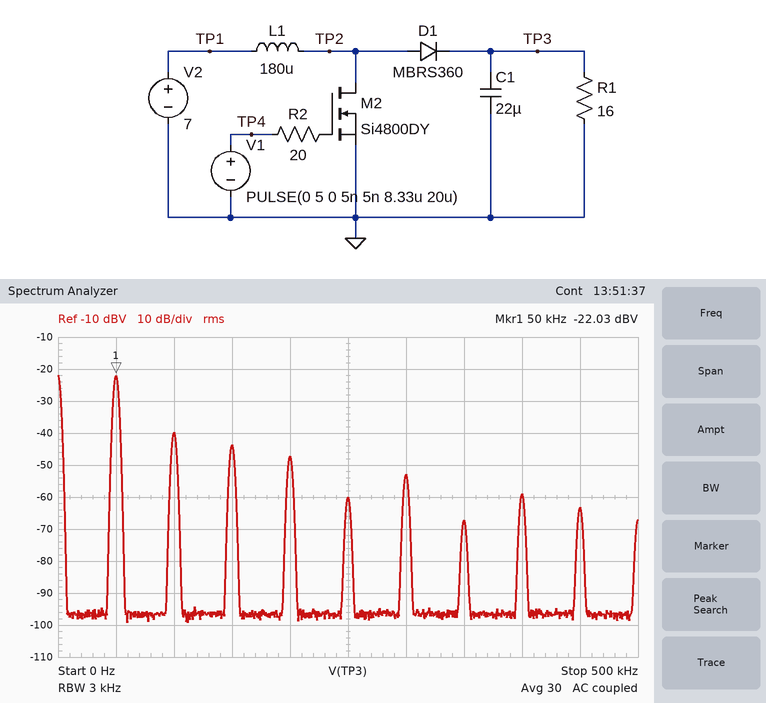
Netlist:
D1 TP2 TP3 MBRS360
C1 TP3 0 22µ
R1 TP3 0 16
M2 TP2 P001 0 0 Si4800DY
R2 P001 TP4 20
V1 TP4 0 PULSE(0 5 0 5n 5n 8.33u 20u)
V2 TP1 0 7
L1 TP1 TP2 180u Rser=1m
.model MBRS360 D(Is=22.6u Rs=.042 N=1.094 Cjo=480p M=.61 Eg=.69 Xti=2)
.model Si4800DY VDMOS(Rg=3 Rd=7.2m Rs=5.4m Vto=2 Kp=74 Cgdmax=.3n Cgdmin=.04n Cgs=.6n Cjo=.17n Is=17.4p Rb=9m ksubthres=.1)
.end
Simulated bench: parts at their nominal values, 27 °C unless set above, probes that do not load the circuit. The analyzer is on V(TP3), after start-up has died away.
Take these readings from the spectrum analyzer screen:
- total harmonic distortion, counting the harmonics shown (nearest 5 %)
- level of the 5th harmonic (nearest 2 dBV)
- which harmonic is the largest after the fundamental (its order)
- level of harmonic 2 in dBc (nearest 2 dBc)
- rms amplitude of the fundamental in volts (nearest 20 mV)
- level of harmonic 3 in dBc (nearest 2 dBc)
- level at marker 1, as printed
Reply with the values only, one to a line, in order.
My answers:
15 %
-60 dBV
2
-18 dBc
80 mV
-22 dBc
-22.03 dBV
